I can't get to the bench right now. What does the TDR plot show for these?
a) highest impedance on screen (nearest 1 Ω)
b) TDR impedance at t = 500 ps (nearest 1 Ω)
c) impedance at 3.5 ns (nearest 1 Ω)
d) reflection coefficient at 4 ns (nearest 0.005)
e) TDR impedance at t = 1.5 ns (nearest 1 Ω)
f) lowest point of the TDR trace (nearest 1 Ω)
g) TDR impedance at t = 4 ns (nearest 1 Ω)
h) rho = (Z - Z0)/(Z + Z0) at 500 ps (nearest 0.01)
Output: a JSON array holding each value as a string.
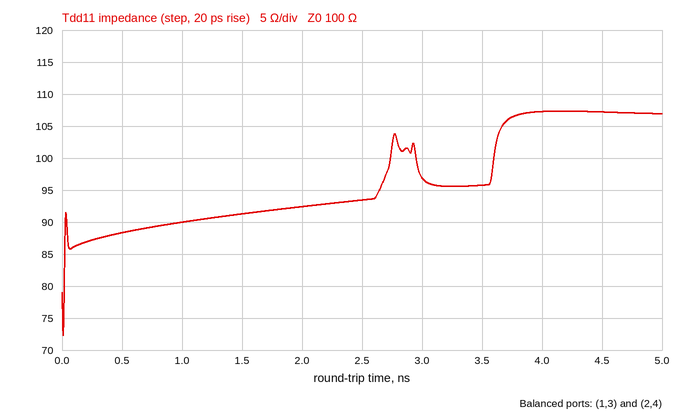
["107 Ω", "88 Ω", "96 Ω", "+0.035", "91 Ω", "72 Ω", "107 Ω", "-0.06"]
